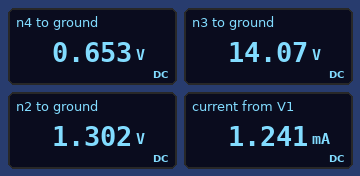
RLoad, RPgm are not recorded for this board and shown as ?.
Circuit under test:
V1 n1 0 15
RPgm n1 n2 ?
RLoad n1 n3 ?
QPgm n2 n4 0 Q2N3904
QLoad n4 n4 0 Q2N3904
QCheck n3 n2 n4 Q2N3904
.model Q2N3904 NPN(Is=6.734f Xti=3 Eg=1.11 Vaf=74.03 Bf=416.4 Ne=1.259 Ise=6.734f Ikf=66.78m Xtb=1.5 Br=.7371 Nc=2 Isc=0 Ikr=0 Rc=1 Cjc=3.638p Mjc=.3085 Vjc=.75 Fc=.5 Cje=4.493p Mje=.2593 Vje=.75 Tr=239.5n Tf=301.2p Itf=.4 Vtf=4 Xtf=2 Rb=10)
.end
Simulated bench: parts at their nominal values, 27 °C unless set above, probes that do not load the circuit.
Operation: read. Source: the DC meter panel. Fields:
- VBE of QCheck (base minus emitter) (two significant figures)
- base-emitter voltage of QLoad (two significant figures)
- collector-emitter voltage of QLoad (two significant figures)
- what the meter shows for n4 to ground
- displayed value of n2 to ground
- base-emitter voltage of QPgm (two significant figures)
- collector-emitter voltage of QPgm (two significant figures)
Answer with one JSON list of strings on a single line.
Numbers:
["650 mV", "650 mV", "650 mV", "0.653 V", "1.302 V", "650 mV", "1.3 V"]
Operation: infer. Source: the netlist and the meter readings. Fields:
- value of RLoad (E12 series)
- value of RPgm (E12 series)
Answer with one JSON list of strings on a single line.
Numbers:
["1.5 kΩ", "22 kΩ"]
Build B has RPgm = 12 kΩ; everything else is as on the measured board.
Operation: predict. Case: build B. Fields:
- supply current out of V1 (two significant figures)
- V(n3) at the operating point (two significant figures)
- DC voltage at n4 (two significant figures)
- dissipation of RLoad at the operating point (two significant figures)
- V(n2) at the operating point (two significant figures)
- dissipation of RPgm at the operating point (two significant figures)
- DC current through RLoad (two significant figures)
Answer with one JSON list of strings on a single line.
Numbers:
["2.3 mA", "13 V", "670 mV", "1.9 mW", "1.3 V", "16 mW", "1.1 mA"]
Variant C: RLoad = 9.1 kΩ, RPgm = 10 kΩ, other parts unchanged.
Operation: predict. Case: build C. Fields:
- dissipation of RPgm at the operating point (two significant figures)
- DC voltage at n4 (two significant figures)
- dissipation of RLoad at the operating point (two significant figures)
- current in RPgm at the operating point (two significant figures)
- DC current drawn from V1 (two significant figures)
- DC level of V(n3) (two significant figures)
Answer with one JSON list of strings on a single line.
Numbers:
["19 mW", "670 mV", "17 mW", "1.4 mA", "2.7 mA", "2.7 V"]
